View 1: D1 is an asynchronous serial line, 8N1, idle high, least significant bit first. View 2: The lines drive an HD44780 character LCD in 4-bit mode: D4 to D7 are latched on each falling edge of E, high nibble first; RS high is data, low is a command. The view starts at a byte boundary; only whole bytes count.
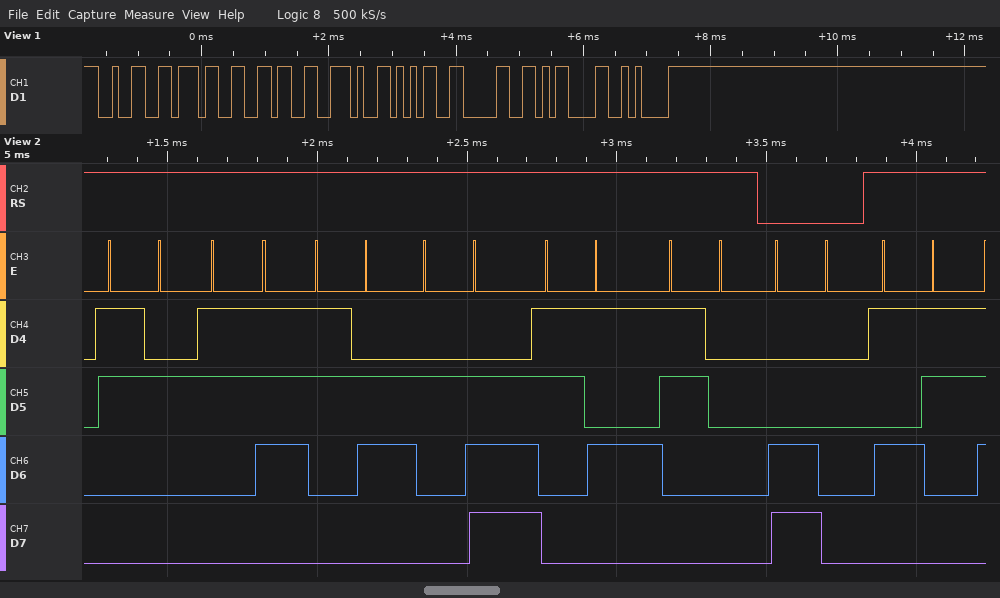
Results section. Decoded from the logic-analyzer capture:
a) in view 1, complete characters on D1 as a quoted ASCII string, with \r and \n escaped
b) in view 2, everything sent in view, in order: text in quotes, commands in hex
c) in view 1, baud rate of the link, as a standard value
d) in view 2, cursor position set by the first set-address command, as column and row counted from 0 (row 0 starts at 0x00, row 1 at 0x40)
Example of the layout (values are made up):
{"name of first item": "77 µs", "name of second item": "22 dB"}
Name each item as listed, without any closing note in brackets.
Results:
{"in view 1, complete characters on D1 as a quoted ASCII string, with \\r and \\n escaped": "\"276.50\\r\\n\"", "in view 2, everything sent in view, in order: text in quotes, commands in hex": "\"276.50\" 0xC0 \"S\"", "in view 1, baud rate of the link, as a standard value": "9600 baud", "in view 2, cursor position set by the first set-address command, as column and row counted from 0": "column 0, row 1"}
